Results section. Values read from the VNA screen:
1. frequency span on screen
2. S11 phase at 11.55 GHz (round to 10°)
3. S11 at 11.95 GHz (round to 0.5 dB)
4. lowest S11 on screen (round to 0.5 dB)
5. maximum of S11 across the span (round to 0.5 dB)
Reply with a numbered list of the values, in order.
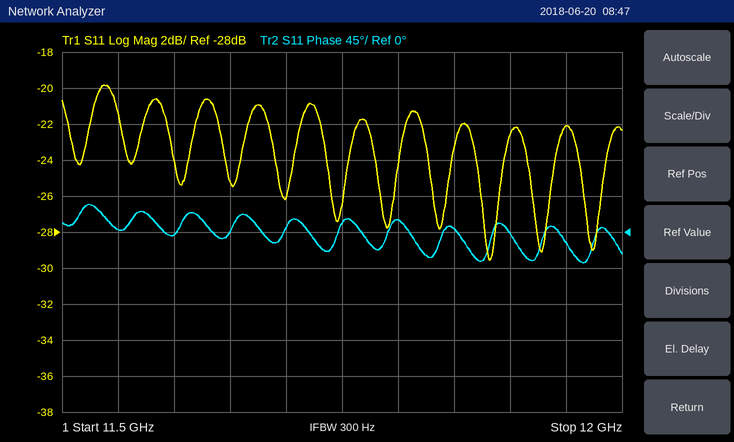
1. 500 MHz
2. 0°
3. -22.0 dB
4. -29.5 dB
5. -20.0 dB
